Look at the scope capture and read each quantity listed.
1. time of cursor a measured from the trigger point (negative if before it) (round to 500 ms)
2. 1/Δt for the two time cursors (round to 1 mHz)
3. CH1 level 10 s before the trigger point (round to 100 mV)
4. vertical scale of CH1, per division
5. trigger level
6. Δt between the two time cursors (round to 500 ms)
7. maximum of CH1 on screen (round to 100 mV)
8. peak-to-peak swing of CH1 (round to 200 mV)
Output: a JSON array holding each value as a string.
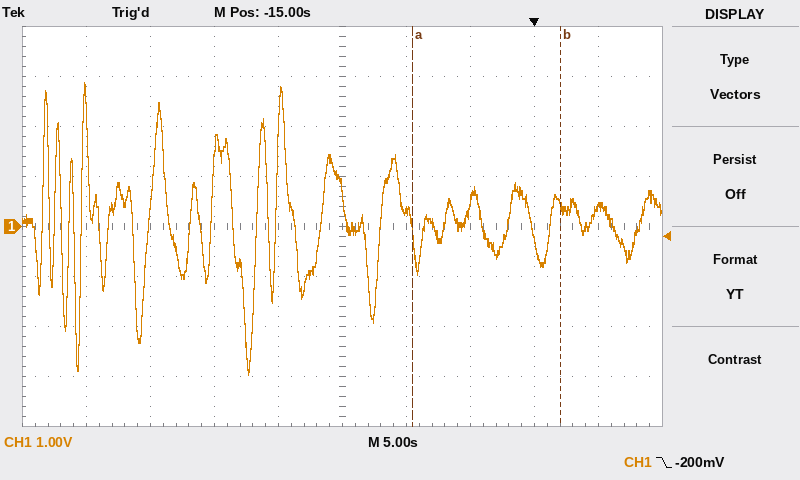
["-9.5 s", "87 mHz", "300 mV", "1 V", "-200 mV", "11.5 s", "2.9 V", "5.8 V"]
